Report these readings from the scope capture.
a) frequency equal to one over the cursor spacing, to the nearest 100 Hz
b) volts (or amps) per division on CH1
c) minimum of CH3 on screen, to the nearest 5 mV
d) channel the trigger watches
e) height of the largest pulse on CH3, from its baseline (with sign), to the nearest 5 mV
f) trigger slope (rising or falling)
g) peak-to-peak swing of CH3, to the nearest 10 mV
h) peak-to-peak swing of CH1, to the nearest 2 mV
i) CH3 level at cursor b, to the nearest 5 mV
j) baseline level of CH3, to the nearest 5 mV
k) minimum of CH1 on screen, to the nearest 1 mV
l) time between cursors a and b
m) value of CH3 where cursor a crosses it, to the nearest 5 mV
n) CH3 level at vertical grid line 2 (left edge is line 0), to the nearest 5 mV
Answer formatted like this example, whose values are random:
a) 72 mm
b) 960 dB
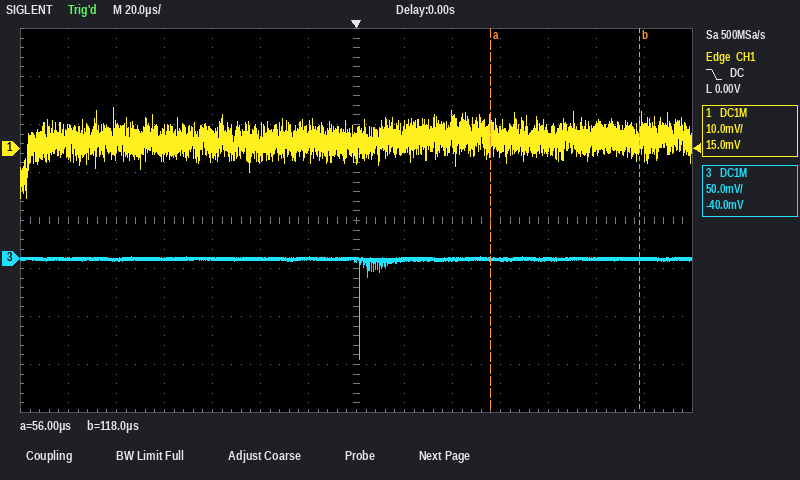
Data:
a) 16.1 kHz
b) 10 mV
c) -105 mV
d) CH1
e) -105 mV
f) falling
g) 110 mV
h) 18 mV
i) 0 mV
j) 0 mV
k) -10 mV
l) 62 µs
m) 0 mV
n) 0 mV
